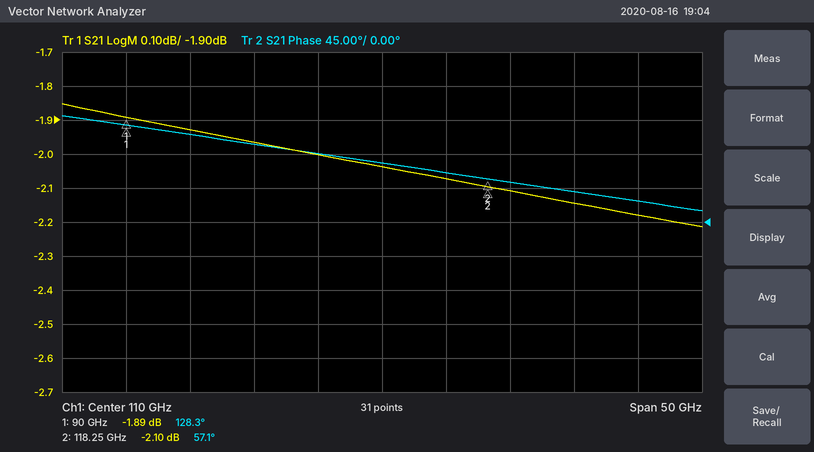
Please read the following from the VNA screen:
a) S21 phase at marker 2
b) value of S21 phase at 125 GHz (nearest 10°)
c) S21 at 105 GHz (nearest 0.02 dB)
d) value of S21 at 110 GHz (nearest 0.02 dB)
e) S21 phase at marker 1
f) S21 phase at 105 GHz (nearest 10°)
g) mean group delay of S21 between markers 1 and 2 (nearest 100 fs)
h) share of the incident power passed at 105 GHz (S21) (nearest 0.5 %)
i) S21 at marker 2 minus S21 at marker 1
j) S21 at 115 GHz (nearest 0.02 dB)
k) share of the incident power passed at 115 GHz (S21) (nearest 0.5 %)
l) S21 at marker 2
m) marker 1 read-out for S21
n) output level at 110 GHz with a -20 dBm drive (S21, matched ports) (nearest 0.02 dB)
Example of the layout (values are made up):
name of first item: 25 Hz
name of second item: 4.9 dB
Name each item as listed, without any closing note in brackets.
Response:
S21 phase at marker 2: 57.1°
value of S21 phase at 125 GHz: 40°
S21 at 105 GHz: -2.00 dB
value of S21 at 110 GHz: -2.04 dB
S21 phase at marker 1: 128.3°
S21 phase at 105 GHz: 90°
mean group delay of S21 between markers 1 and 2: 7.0 ps
share of the incident power passed at 105 GHz (S21): 63.0 %
S21 at marker 2 minus S21 at marker 1: -0.21 dB
S21 at 115 GHz: -2.08 dB
share of the incident power passed at 115 GHz (S21): 62.0 %
S21 at marker 2: -2.10 dB
marker 1 read-out for S21: -1.89 dB
output level at 110 GHz with a -20 dBm drive (S21, matched ports): -22.04 dBm
